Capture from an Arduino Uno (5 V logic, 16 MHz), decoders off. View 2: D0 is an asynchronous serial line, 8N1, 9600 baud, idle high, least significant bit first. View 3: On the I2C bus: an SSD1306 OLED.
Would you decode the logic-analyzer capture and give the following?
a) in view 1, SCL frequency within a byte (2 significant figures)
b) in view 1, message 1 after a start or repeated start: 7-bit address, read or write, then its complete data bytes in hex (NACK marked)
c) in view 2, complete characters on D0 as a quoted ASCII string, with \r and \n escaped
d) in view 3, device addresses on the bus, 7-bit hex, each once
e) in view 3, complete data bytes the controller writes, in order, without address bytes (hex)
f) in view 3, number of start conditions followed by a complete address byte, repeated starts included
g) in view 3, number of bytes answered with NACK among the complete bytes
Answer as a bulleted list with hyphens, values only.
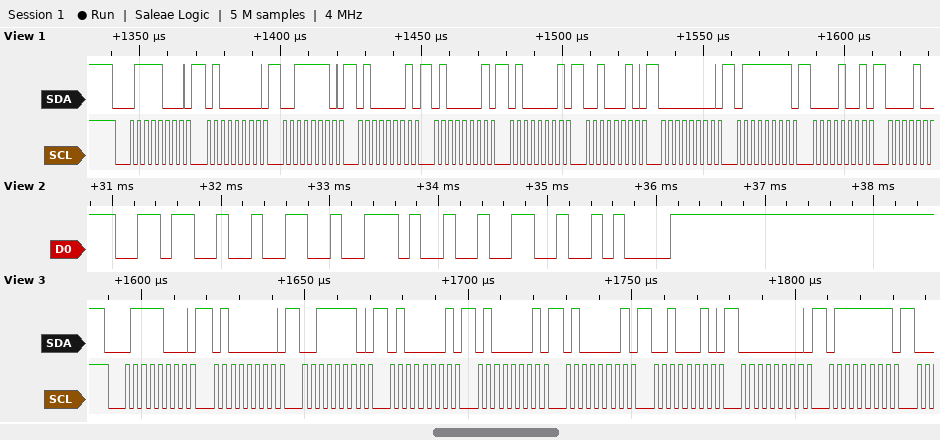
- 400 kHz
- 0x3C write: 40 3E 41 41 41 22 00 7F 09
- "62.2\n"
- 0x3C
- 40 3E 41 41 41 22 00 7F
- 1
- 0
